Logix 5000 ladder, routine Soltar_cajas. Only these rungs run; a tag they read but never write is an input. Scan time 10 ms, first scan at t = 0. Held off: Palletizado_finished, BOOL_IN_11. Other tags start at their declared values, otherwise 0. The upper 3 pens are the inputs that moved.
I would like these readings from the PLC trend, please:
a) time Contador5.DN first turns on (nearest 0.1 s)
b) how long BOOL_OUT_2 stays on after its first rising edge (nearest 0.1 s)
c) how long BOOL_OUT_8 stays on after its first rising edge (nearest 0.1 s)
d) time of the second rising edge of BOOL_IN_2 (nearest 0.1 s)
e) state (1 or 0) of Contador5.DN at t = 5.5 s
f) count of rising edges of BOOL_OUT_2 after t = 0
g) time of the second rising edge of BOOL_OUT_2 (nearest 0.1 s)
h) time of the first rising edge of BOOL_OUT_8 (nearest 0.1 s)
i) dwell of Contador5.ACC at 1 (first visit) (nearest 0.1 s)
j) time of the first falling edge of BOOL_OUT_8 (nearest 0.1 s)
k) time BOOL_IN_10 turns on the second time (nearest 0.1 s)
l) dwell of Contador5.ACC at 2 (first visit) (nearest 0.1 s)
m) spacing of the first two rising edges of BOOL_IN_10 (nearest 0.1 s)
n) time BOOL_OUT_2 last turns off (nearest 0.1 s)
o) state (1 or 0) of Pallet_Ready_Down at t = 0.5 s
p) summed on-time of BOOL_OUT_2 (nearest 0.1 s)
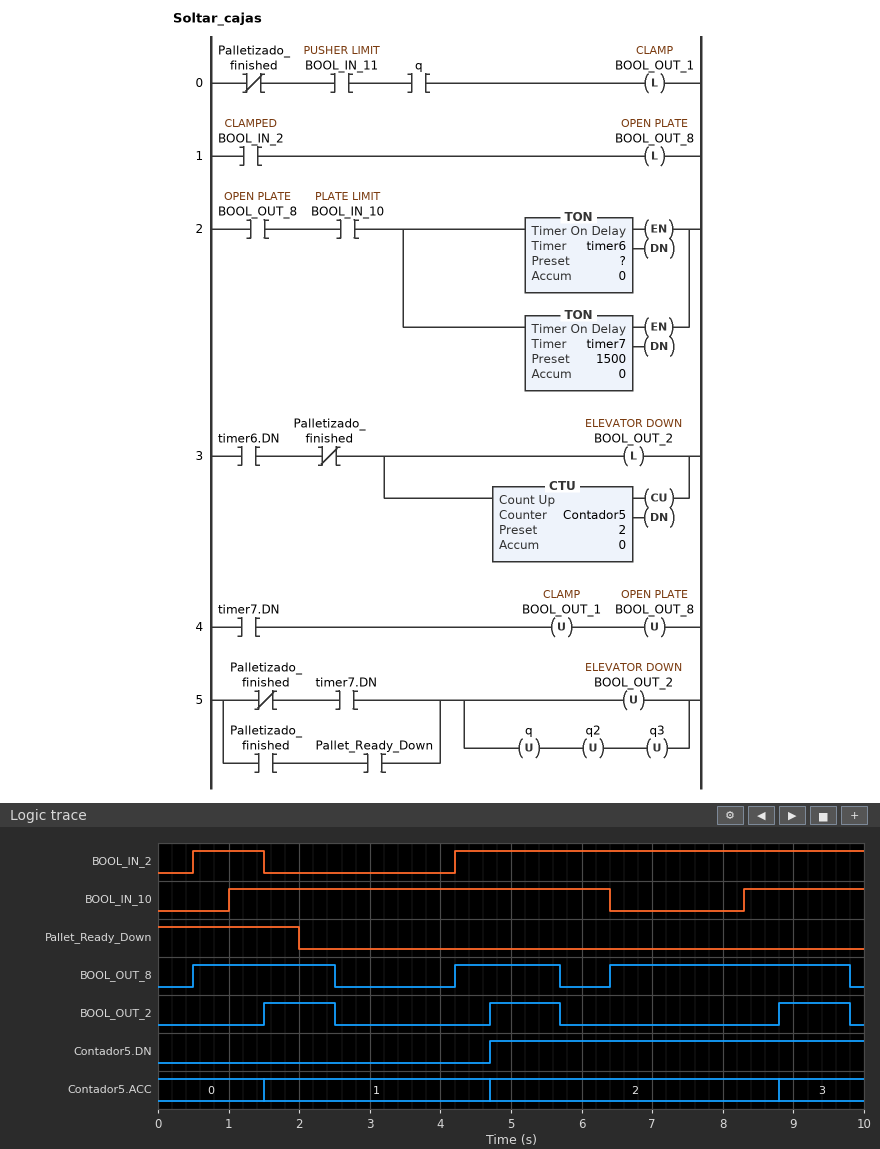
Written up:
4.7 s
1.0 s
2.0 s
4.2 s
1
3
4.7 s
0.5 s
3.2 s
2.5 s
8.3 s
4.1 s
7.3 s
9.8 s
1
3.0 s
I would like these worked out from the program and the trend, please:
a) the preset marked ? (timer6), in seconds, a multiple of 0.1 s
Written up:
0.5 s
